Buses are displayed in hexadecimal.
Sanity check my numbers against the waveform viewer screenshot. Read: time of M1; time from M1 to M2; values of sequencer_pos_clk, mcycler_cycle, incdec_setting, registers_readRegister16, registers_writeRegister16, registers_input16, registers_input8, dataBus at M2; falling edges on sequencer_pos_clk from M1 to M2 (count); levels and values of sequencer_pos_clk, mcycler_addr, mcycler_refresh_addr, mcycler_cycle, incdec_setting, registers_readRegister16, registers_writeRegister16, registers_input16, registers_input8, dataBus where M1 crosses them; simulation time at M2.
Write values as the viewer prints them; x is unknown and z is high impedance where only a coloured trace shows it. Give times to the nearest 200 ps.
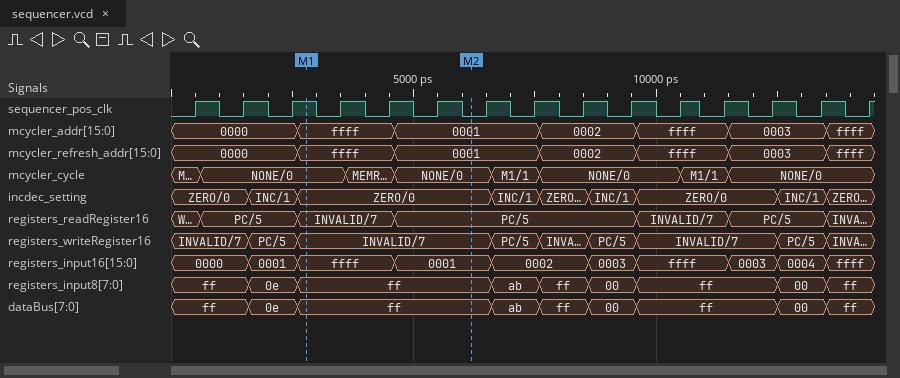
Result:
2800 ps
3400 ps
sequencer_pos_clk=0, mcycler_cycle=NONE/0, incdec_setting=ZERO/0, registers_readRegister16=PC/5, registers_writeRegister16=INVALID/7, registers_input16=0001, registers_input8=ff, dataBus=ff
4
sequencer_pos_clk=1, mcycler_addr=ffff, mcycler_refresh_addr=ffff, mcycler_cycle=NONE/0, incdec_setting=ZERO/0, registers_readRegister16=INVALID/7, registers_writeRegister16=INVALID/7, registers_input16=ffff, registers_input8=ff, dataBus=ff
6200 ps
